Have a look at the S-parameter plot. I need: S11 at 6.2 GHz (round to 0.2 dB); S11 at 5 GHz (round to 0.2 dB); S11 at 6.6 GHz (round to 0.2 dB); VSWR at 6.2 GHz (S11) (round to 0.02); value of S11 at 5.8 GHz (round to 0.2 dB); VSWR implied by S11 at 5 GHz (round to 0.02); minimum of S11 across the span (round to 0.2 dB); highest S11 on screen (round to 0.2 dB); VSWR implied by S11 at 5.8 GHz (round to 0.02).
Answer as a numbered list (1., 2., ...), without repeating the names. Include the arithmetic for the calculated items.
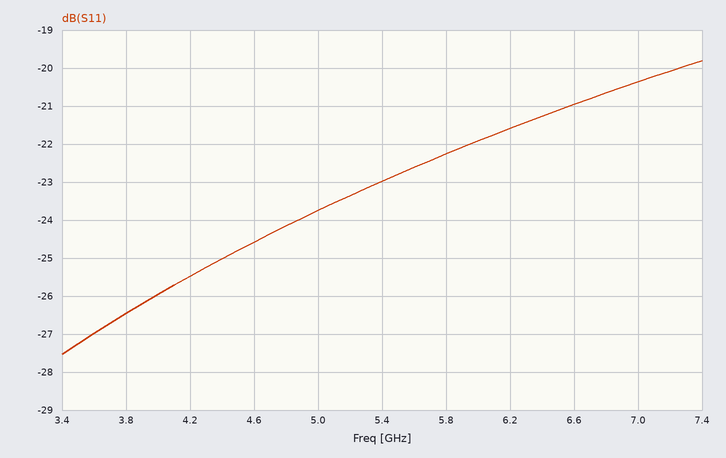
1. -21.6 dB
2. -23.8 dB
3. -21.0 dB
4. |Γ| = 10^(-21.6/20) = 0.0832; VSWR = (1 + 0.0832)/(1 − 0.0832) ≈ 1.18
5. -22.2 dB
6. |Γ| = 10^(-23.8/20) = 0.0646; VSWR = (1 + 0.0646)/(1 − 0.0646) ≈ 1.14
7. -27.6 dB
8. -19.8 dB
9. |Γ| = 10^(-22.2/20) = 0.0776; VSWR = (1 + 0.0776)/(1 − 0.0776) ≈ 1.17, so 1.16 to the nearest 0.02
